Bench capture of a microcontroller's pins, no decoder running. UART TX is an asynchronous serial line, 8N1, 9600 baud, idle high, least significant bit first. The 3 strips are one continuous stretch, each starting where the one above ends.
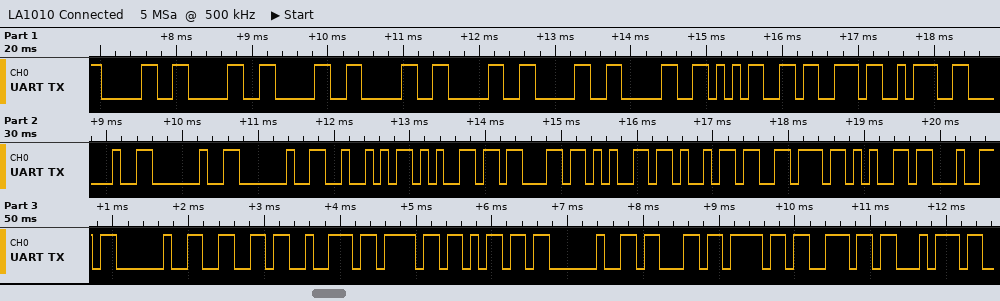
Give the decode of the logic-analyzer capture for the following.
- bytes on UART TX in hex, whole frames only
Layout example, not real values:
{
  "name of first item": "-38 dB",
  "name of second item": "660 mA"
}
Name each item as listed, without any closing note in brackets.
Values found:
{
  "bytes on UART TX in hex, whole frames only": "30 30 30 30 30 30 30 35 73 3A 20 20 20 52 65 63 65 69 76 65 64 20 66 72 6F 6D 20 63 6F 6E 74"
}
